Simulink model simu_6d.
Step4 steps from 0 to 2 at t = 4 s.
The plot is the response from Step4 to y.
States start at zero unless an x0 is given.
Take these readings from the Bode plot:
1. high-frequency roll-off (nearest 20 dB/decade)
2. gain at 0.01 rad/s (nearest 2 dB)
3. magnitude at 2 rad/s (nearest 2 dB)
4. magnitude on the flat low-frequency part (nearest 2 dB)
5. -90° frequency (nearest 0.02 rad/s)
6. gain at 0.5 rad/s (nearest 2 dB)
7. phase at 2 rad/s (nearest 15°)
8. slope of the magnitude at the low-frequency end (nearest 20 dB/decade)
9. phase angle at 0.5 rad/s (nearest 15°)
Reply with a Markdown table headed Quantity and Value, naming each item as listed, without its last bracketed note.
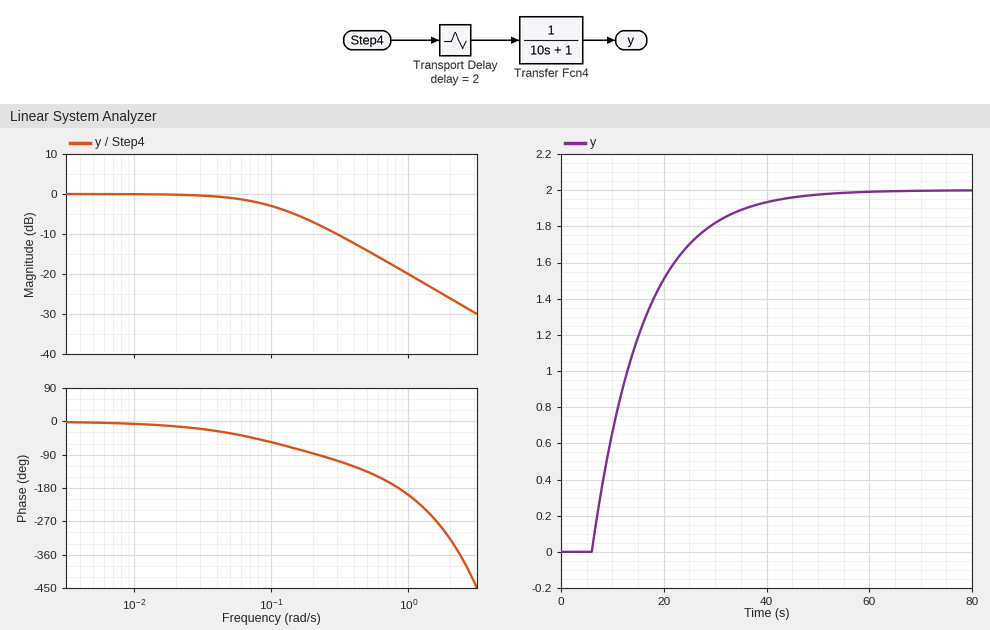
| Quantity | Value |
|---|---|
| high-frequency roll-off | -20 dB/decade |
| gain at 0.01 rad/s | 0 dB |
| magnitude at 2 rad/s | -26 dB |
| magnitude on the flat low-frequency part | 0 dB |
| -90° frequency | 0.22 rad/s |
| gain at 0.5 rad/s | -14 dB |
| phase at 2 rad/s | -315° |
| slope of the magnitude at the low-frequency end | 0 dB/decade |
| phase angle at 0.5 rad/s | -135° |
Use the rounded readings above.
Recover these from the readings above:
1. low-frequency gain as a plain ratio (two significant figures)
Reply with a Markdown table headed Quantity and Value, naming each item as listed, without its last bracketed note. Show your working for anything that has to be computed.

| Quantity | Value |
|---|---|
| low-frequency gain as a plain ratio | 10^(0 / 20) = 1.0 |
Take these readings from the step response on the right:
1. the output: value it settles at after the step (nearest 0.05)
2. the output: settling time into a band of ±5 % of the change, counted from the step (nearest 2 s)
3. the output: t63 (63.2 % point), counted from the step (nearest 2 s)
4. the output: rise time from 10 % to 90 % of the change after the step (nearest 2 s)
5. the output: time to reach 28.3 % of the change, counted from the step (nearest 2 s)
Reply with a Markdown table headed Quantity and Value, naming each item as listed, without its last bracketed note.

| Quantity | Value |
|---|---|
| the output: value it settles at after the step | 2.00 |
| the output: settling time into a band of ±5 % of the change, counted from the step | 32 s |
| the output: t63 (63.2 % point), counted from the step | 12 s |
| the output: rise time from 10 % to 90 % of the change after the step | 22 s |
| the output: time to reach 28.3 % of the change, counted from the step | 6 s |
